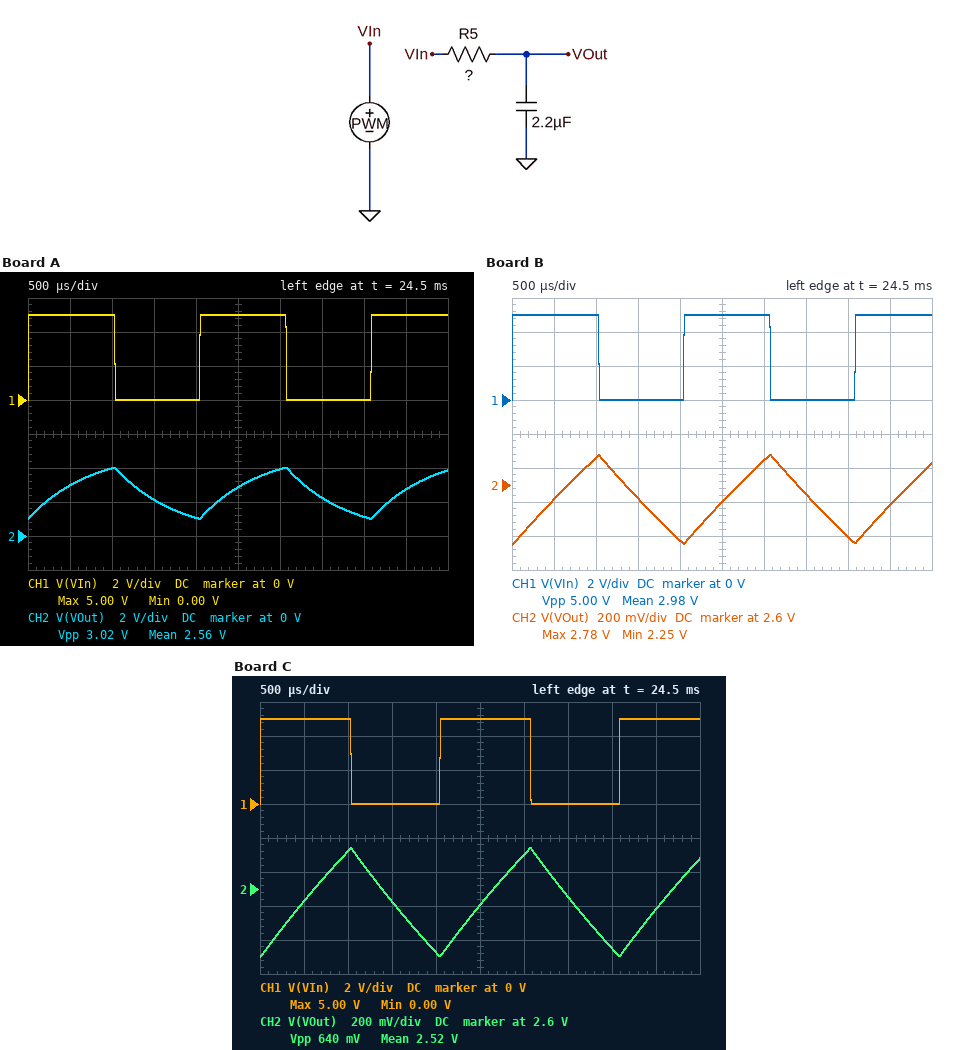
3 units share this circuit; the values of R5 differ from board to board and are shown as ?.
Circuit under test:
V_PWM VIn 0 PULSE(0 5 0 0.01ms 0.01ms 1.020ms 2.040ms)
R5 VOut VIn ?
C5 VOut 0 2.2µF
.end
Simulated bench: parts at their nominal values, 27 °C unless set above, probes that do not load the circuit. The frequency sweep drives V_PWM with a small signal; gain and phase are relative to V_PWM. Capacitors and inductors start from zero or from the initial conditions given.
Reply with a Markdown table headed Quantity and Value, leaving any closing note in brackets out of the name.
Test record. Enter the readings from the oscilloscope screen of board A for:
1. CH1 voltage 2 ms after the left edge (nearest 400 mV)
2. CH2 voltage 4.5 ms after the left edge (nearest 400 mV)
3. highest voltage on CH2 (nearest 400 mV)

| Quantity | Value |
|---|---|
| CH1 voltage 2 ms after the left edge | 0 V |
| CH2 voltage 4.5 ms after the left edge | 2.8 V |
| highest voltage on CH2 | 4.0 V |
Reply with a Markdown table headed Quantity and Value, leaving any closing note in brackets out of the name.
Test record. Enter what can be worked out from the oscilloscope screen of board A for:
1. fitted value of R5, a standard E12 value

| Quantity | Value |
|---|---|
| fitted value of R5, a standard E12 value | 330 Ω |
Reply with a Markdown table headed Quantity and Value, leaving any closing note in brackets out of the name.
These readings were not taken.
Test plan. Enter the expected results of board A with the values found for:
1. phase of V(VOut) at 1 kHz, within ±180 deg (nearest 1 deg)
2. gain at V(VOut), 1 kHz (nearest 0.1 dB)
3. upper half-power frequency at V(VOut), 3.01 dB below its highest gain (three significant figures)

| Quantity | Value |
|---|---|
| phase of V(VOut) at 1 kHz, within ±180 deg | -78 deg |
| gain at V(VOut), 1 kHz | -13.4 dB |
| upper half-power frequency at V(VOut), 3.01 dB below its highest gain | 219 Hz |
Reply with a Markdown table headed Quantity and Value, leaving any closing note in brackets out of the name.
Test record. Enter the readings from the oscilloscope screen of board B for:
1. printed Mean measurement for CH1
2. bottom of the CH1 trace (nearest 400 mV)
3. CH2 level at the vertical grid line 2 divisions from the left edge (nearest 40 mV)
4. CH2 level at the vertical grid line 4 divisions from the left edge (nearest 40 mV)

| Quantity | Value |
|---|---|
| printed Mean measurement for CH1 | 2.98 V |
| bottom of the CH1 trace | 0 V |
| CH2 level at the vertical grid line 2 divisions from the left edge | 2.76 V |
| CH2 level at the vertical grid line 4 divisions from the left edge | 2.28 V |
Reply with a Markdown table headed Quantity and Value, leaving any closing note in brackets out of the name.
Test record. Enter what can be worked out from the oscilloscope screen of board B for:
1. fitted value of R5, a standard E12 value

| Quantity | Value |
|---|---|
| fitted value of R5, a standard E12 value | 2.2 kΩ |
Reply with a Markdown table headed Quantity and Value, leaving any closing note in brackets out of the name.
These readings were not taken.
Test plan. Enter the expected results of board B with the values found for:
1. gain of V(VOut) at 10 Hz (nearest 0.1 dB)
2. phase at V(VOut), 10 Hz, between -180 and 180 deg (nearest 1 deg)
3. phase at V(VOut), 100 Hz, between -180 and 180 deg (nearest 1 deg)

| Quantity | Value |
|---|---|
| gain of V(VOut) at 10 Hz | -0.4 dB |
| phase at V(VOut), 10 Hz, between -180 and 180 deg | -17 deg |
| phase at V(VOut), 100 Hz, between -180 and 180 deg | -72 deg |
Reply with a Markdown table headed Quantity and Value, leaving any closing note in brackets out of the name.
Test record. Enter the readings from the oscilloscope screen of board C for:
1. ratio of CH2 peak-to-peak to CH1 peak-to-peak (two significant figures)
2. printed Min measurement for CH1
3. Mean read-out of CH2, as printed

| Quantity | Value |
|---|---|
| ratio of CH2 peak-to-peak to CH1 peak-to-peak | 0.13 |
| printed Min measurement for CH1 | 0.00 V |
| Mean read-out of CH2, as printed | 2.52 V |
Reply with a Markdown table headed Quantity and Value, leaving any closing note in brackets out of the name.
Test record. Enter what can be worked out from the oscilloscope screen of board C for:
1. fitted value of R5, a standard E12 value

| Quantity | Value |
|---|---|
| fitted value of R5, a standard E12 value | 1.8 kΩ |
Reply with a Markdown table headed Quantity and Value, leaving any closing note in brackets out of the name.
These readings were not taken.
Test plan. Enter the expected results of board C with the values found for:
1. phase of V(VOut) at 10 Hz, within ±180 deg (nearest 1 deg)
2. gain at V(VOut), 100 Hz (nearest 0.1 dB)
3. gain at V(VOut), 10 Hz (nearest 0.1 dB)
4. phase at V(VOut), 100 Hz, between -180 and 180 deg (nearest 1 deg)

| Quantity | Value |
|---|---|
| phase of V(VOut) at 10 Hz, within ±180 deg | -14 deg |
| gain at V(VOut), 100 Hz | -8.6 dB |
| gain at V(VOut), 10 Hz | -0.3 dB |
| phase at V(VOut), 100 Hz, between -180 and 180 deg | -68 deg |
